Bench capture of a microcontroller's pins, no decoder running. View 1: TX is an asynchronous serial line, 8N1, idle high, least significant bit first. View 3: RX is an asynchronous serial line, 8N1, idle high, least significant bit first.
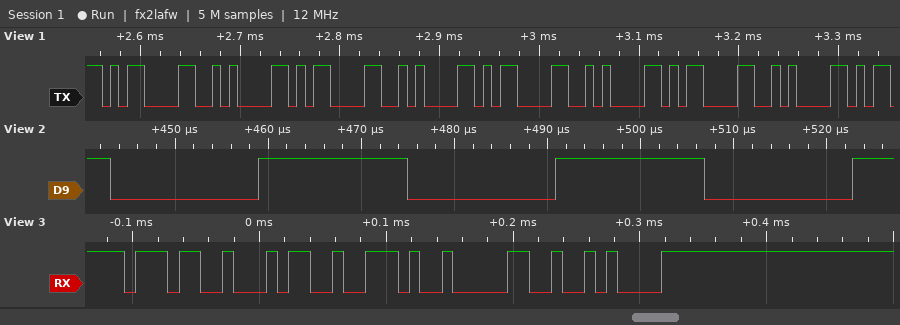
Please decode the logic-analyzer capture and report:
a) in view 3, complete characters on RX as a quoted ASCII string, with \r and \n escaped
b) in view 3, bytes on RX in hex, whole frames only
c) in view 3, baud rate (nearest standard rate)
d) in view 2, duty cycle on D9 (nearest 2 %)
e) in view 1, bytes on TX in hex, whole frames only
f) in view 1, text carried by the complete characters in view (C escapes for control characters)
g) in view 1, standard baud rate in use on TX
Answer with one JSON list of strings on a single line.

["\"74.0\\n\"", "37 34 2E 30 0A", "115200 baud", "50 %", "0x0D 0x0A 0x0D 0x0A 0x0D 0x0A 0x0D 0x0A", "\"\\r\\n\\r\\n\\r\\n\\r\\n\"", "115200 baud"]
